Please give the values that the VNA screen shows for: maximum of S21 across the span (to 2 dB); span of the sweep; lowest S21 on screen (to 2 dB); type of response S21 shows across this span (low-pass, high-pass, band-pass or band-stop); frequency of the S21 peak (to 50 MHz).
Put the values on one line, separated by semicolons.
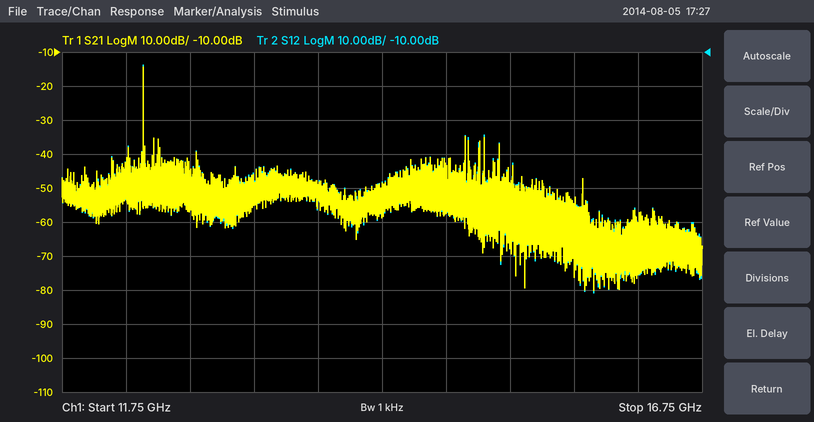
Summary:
-14 dB; 5 GHz; -80 dB; band-pass; 12.40 GHz
